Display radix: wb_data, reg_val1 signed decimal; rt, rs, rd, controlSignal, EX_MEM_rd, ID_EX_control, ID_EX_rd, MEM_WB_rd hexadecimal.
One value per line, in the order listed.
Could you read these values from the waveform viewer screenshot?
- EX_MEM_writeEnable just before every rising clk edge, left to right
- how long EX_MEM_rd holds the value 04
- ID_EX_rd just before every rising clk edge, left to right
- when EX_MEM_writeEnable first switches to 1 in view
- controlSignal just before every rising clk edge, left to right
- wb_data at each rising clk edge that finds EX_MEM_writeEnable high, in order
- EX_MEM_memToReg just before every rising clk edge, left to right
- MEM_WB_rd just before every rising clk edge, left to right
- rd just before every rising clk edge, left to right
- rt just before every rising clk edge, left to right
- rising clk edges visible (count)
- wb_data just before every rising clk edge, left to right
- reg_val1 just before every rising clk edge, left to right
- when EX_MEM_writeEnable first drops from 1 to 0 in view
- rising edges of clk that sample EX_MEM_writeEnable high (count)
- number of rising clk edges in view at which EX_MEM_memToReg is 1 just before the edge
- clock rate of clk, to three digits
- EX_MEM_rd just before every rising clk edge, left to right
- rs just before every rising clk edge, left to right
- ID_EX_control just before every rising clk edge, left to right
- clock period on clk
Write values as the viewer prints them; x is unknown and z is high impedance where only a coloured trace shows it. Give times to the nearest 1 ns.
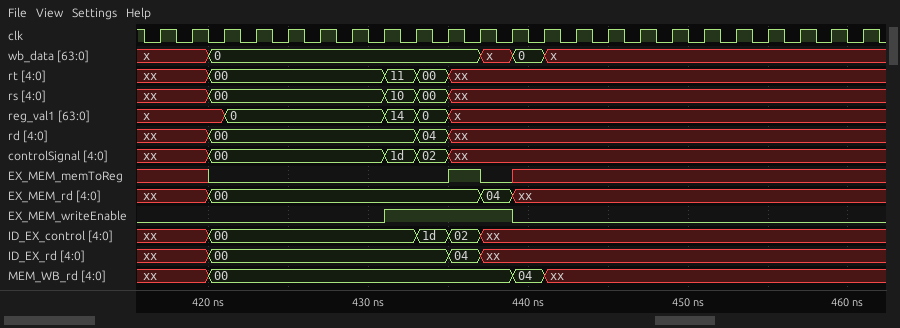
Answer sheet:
0 0 0 0 0 0 0 0 1 1 1 1 0 0 0 0 0 0 0 0 0 0 0
2 ns
xx, xx, 00, 00, 00, 00, 00, 00, 00, 00, 04, xx, xx, xx, xx, xx, xx, xx, xx, xx, xx, xx, xx
431 ns
xx, xx, 00, 00, 00, 00, 00, 00, 1d, 02, xx, xx, xx, xx, xx, xx, xx, xx, xx, xx, xx, xx, xx
0, 0, 0, x
x x 0 0 0 0 0 0 0 0 1 0 x x x x x x x x x x x
xx, xx, 00, 00, 00, 00, 00, 00, 00, 00, 00, 00, 04, xx, xx, xx, xx, xx, xx, xx, xx, xx, xx
xx, xx, 00, 00, 00, 00, 00, 00, 00, 04, xx, xx, xx, xx, xx, xx, xx, xx, xx, xx, xx, xx, xx
xx, xx, 00, 00, 00, 00, 00, 00, 11, 00, xx, xx, xx, xx, xx, xx, xx, xx, xx, xx, xx, xx, xx
23
x, x, 0, 0, 0, 0, 0, 0, 0, 0, 0, x, 0, x, x, x, x, x, x, x, x, x, x
x, x, x, 0, 0, 0, 0, 0, 14, 0, x, x, x, x, x, x, x, x, x, x, x, x, x
439 ns
4
1
500 MHz
xx, xx, 00, 00, 00, 00, 00, 00, 00, 00, 00, 04, xx, xx, xx, xx, xx, xx, xx, xx, xx, xx, xx
xx, xx, 00, 00, 00, 00, 00, 00, 10, 00, xx, xx, xx, xx, xx, xx, xx, xx, xx, xx, xx, xx, xx
xx, xx, 00, 00, 00, 00, 00, 00, 00, 1d, 02, xx, xx, xx, xx, xx, xx, xx, xx, xx, xx, xx, xx
2 ns
